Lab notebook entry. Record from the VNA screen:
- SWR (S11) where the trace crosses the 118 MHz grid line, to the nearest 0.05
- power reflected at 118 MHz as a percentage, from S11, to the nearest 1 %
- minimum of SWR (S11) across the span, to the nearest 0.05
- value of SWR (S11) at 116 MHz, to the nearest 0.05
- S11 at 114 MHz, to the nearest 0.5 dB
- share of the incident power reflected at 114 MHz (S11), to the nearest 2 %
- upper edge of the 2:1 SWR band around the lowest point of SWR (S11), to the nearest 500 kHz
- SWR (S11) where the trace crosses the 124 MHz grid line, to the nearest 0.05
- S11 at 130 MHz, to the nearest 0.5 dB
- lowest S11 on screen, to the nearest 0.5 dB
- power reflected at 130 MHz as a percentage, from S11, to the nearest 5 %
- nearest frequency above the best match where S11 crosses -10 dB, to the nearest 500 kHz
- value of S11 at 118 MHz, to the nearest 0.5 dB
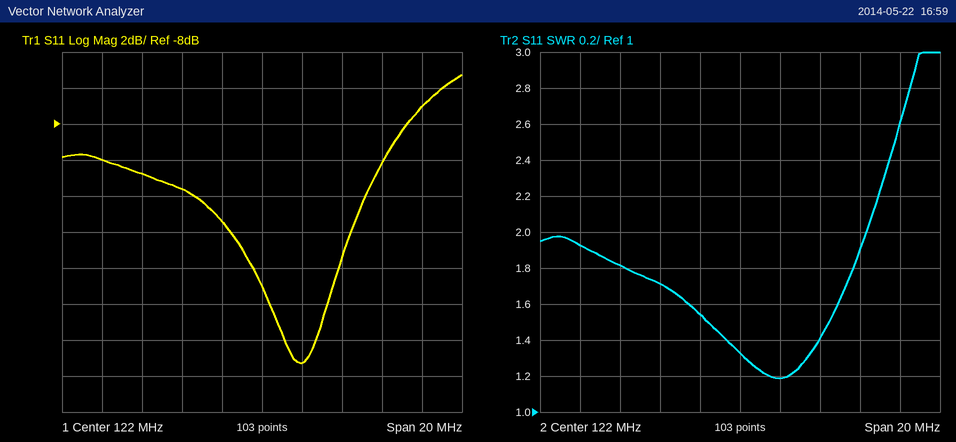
1.70
7 %
1.20
1.80
-10.0 dB
10 %
128.5 MHz
1.20
-7.0 dB
-21.5 dB
20 %
128.0 MHz
-11.5 dB
